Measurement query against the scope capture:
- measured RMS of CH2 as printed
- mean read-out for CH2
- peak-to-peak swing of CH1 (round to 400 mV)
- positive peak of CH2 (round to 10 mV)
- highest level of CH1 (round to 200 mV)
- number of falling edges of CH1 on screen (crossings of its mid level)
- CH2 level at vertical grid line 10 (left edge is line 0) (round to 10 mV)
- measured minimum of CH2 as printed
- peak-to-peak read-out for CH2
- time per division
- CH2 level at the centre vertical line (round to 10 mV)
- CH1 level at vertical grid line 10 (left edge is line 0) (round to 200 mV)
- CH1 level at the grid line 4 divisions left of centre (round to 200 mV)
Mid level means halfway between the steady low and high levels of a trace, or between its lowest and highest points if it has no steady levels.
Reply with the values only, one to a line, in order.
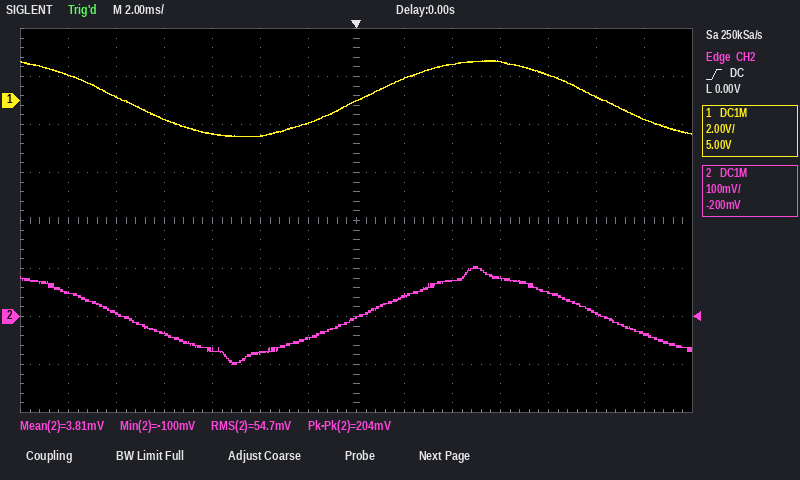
54.7 mV
3.81 mV
3.2 V
100 mV
1.6 V
2
80 mV
-100 mV
204 mV
2 ms
0 mV
1.6 V
-800 mV
